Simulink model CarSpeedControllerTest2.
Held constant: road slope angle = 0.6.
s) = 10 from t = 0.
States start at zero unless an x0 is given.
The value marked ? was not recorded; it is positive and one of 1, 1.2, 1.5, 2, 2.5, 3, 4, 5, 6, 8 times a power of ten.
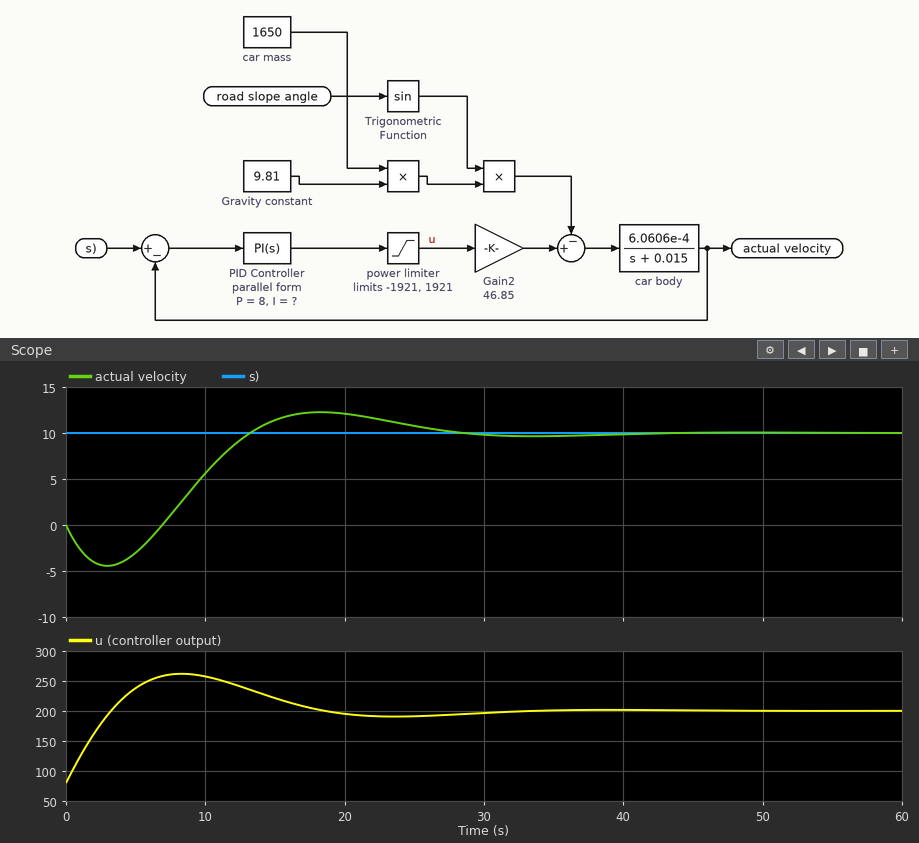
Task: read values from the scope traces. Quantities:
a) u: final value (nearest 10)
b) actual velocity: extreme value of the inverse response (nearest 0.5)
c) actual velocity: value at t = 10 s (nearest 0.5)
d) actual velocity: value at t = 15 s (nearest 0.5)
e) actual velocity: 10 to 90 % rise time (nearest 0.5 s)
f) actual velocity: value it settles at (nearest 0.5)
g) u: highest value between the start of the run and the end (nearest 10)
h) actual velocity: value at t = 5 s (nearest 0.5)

200
-4.5
5.5
11.5
5.0 s
10.0
260
-3.0
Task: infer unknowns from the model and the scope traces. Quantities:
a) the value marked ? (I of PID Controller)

2
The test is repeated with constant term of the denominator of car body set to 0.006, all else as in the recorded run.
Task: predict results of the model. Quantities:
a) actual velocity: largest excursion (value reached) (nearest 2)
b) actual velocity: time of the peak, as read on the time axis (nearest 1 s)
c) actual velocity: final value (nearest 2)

12
18 s
10
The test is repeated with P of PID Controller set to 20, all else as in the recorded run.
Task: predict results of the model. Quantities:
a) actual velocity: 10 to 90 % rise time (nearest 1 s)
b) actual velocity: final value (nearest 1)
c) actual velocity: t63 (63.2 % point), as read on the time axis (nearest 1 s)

19 s
10
10 s
